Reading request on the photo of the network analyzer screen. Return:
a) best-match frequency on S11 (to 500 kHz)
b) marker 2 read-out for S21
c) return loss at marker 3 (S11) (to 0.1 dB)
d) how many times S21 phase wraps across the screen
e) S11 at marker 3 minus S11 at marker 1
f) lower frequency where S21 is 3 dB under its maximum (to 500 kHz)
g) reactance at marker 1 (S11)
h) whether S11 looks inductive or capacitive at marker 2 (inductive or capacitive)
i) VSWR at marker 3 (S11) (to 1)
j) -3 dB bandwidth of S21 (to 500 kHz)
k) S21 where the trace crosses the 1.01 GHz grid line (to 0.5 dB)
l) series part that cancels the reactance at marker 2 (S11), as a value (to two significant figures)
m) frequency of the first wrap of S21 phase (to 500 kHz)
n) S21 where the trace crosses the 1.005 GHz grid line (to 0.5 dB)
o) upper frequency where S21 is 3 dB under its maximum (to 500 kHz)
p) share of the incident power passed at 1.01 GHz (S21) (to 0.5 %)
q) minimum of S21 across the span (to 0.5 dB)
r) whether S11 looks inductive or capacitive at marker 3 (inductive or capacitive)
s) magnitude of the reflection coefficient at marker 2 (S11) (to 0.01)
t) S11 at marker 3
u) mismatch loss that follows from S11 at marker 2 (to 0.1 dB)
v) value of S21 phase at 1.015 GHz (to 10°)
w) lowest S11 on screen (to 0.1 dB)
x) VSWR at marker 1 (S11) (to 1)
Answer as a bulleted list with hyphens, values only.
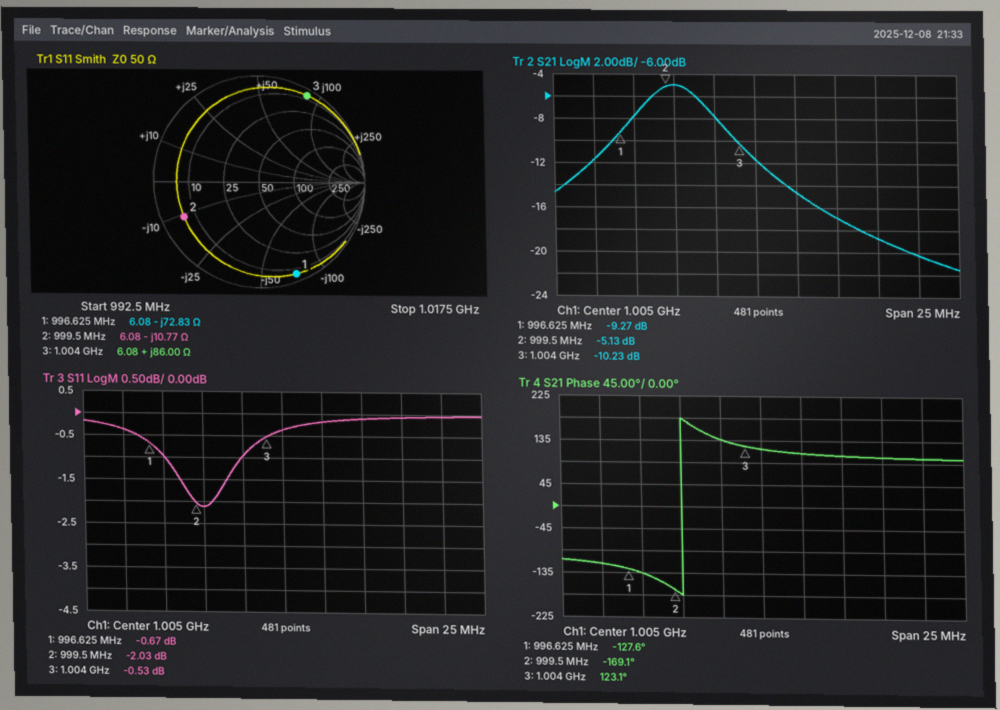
- 1.0000 GHz
- -5.13 dB
- 0.5 dB
- 1
- 0.14 dB
- 997.5 MHz
- -72.83 Ω
- capacitive
- 33
- 5.0 MHz
- -17.0 dB
- 1.7 nH
- 1.0000 GHz
- -11.5 dB
- 1.0025 GHz
- 2.0 %
- -21.5 dB
- inductive
- 0.79
- -0.53 dB
- 4.3 dB
- 100°
- -2.1 dB
- 26
